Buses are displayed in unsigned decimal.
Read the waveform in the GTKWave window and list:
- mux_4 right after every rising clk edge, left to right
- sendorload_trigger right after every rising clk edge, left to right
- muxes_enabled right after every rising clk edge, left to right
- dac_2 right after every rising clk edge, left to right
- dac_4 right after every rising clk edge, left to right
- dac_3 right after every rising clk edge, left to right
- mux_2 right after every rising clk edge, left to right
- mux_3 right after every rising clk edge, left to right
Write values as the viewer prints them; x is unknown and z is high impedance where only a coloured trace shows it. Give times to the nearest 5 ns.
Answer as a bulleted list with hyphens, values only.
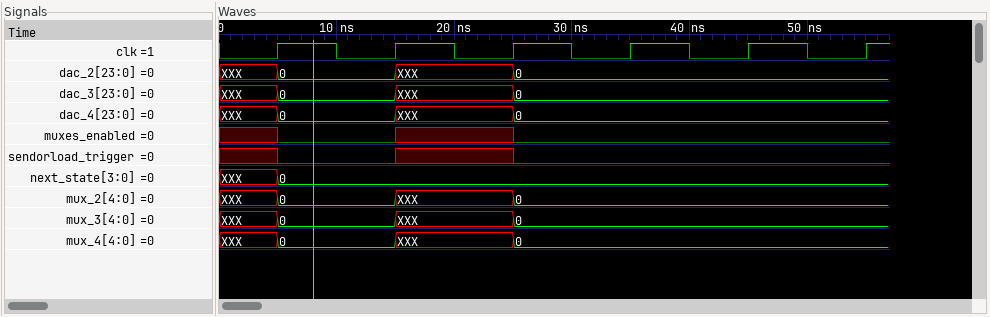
- 0, XXX, 0, 0, 0, 0
- 0 x 0 0 0 0
- 0 x 0 0 0 0
- 0, XXX, 0, 0, 0, 0
- 0, XXX, 0, 0, 0, 0
- 0, XXX, 0, 0, 0, 0
- 0, XXX, 0, 0, 0, 0
- 0, XXX, 0, 0, 0, 0
